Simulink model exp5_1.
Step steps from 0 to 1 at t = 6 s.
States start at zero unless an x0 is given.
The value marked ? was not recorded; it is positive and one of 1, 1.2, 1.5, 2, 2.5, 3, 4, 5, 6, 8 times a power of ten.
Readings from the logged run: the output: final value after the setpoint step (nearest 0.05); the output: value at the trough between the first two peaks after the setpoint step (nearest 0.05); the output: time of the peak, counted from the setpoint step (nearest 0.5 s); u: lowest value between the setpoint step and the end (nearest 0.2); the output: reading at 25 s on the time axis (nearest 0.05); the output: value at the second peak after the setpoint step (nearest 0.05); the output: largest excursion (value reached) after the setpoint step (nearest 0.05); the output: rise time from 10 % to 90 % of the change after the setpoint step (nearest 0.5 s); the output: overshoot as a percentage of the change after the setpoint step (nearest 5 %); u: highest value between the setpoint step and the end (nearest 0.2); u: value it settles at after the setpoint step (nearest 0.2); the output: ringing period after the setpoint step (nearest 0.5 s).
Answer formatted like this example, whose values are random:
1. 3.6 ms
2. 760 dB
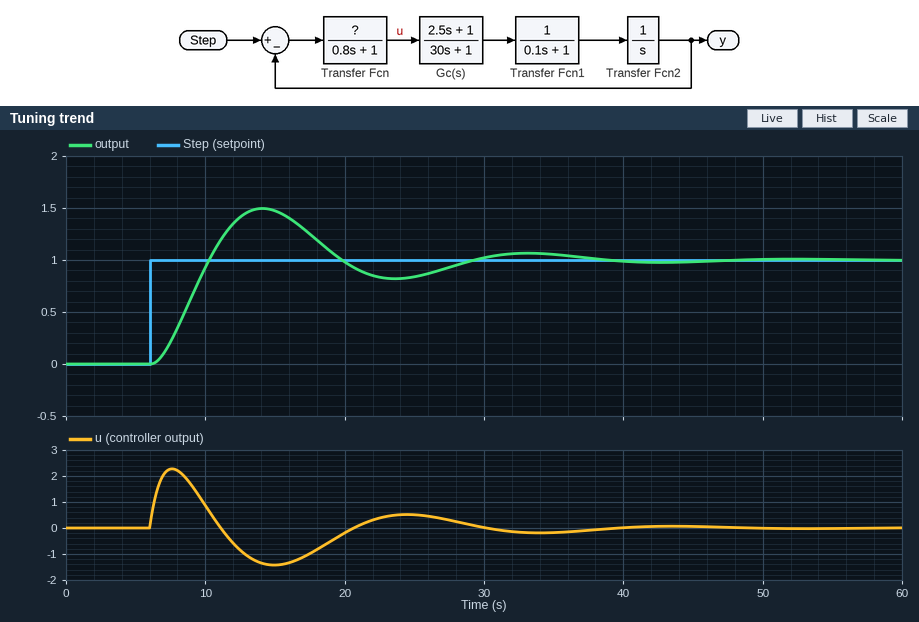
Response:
1. 1.00
2. 0.80
3. 8.0 s
4. -1.4
5. 0.85
6. 1.05
7. 1.50
8. 3.0 s
9. 50 %
10. 2.2
11. 0.0
12. 19.0 s
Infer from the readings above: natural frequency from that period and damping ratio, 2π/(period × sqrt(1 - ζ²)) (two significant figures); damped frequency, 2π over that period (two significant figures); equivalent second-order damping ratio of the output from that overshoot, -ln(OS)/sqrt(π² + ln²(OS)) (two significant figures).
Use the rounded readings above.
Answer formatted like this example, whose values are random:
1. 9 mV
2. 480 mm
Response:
1. 0.34 rad/s
2. 0.33 rad/s
3. 0.22
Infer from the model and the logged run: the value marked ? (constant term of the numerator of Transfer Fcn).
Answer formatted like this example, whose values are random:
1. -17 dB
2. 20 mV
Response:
1. 3
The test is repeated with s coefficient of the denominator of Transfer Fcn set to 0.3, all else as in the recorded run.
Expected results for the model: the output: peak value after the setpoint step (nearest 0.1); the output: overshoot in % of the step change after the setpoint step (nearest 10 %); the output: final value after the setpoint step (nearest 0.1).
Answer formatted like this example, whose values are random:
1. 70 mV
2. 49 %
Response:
1. 1.4
2. 40 %
3. 1.0
